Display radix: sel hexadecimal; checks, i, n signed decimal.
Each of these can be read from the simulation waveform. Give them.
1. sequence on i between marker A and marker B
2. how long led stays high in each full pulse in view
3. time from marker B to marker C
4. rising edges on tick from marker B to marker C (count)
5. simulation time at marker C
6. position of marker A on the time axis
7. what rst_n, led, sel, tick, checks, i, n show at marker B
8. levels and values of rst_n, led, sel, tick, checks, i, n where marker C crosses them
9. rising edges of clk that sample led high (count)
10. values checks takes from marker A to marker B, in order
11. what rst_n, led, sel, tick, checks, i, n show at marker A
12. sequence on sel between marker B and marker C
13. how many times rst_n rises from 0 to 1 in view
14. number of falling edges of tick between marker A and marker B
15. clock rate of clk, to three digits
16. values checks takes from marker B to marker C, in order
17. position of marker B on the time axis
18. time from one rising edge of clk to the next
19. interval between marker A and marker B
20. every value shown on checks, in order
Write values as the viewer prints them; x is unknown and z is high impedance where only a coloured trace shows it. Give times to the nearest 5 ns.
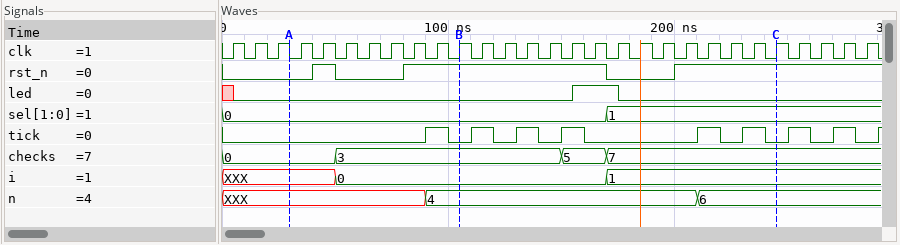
XXX, 0
20 ns
140 ns
5
245 ns
30 ns
rst_n=1, led=0, sel=0, tick=0, checks=3, i=0, n=4
rst_n=1, led=0, sel=1, tick=0, checks=7, i=1, n=6
2
0, 3
rst_n=0, led=0, sel=0, tick=0, checks=0, i=XXX, n=XXX
0, 1
3
1
100 MHz
3, 5, 7
105 ns
10 ns
75 ns
0, 3, 5, 7
